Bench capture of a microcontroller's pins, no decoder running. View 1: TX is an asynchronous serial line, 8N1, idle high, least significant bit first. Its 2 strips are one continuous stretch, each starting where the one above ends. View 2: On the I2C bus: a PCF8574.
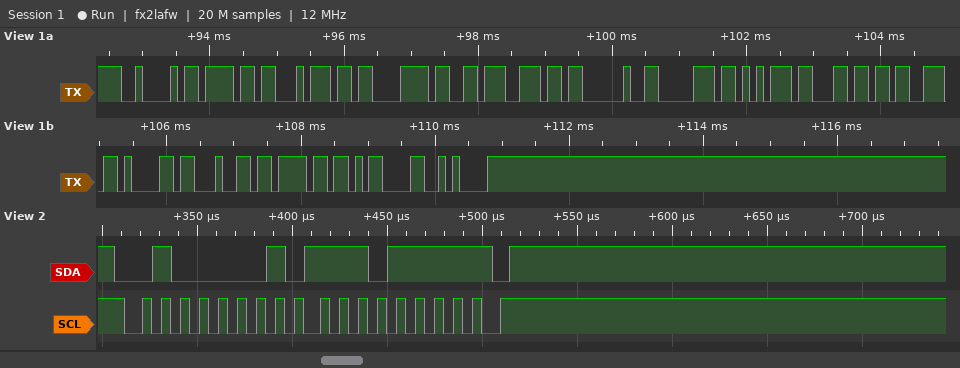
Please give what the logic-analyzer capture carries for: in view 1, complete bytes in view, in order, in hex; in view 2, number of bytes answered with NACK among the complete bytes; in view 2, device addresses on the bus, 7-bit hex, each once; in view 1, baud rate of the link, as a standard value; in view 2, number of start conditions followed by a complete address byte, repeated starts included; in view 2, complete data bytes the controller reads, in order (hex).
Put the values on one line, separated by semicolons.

0x42 0x6F 0x74 0xC3 0xB3 0x6E 0x20 0x70 0x75 0x6C 0x73 0x61 0x64 0x6F 0x0D 0x0A; 1; 0x20; 9600 baud; 1; EF
